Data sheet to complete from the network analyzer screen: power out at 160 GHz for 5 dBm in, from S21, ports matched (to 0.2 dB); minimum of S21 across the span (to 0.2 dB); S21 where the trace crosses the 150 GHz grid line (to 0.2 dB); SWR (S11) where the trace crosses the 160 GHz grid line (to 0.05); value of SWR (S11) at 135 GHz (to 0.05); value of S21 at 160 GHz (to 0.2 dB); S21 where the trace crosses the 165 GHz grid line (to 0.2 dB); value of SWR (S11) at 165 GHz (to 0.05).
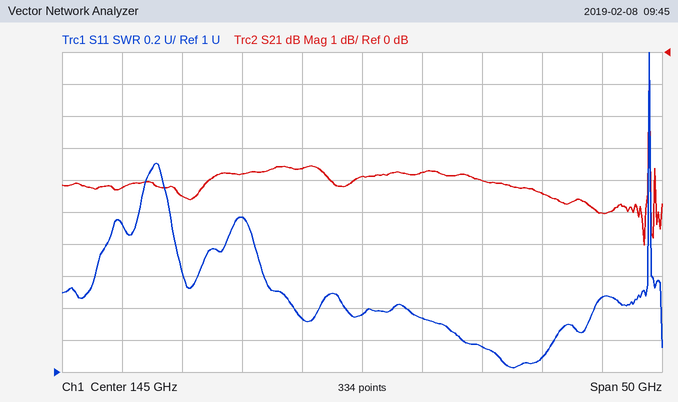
0.6 dBm
-6.0 dB
-3.8 dB
1.10
1.95
-4.4 dB
-5.0 dB
1.45
